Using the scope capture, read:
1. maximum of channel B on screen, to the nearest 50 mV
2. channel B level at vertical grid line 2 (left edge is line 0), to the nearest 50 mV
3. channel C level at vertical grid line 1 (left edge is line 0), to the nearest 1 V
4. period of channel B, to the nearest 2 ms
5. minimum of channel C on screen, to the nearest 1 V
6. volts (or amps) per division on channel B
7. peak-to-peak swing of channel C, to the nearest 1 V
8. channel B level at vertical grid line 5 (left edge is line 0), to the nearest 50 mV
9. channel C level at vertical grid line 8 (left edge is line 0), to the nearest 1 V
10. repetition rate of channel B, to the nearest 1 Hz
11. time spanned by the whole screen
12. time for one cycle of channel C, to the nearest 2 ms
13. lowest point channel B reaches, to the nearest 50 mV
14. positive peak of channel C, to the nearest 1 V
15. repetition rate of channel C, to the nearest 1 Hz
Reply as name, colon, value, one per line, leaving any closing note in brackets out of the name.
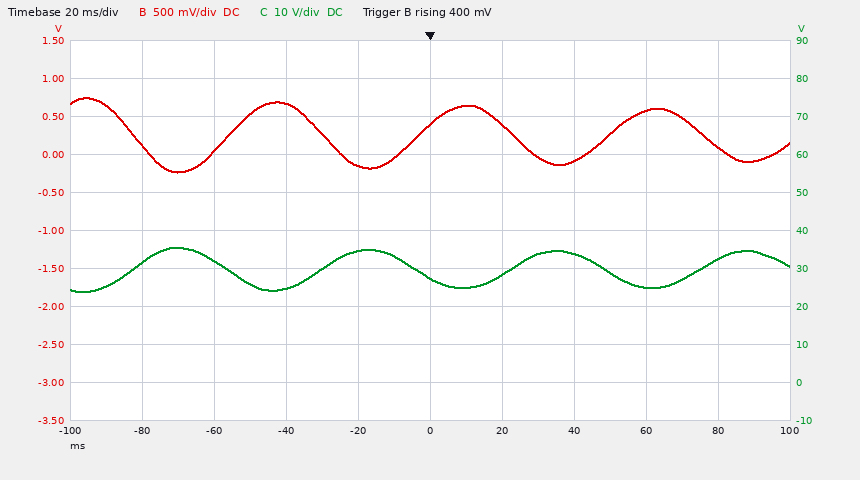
maximum of channel B on screen, to the nearest 50 mV: 750 mV
channel B level at vertical grid line 2 (left edge is line 0), to the nearest 50 mV: 50 mV
channel C level at vertical grid line 1 (left edge is line 0), to the nearest 1 V: 32 V
period of channel B, to the nearest 2 ms: 52 ms
minimum of channel C on screen, to the nearest 1 V: 24 V
volts (or amps) per division on channel B: 500 mV
peak-to-peak swing of channel C, to the nearest 1 V: 12 V
channel B level at vertical grid line 5 (left edge is line 0), to the nearest 50 mV: 400 mV
channel C level at vertical grid line 8 (left edge is line 0), to the nearest 1 V: 25 V
repetition rate of channel B, to the nearest 1 Hz: 19 Hz
time spanned by the whole screen: 200 ms
time for one cycle of channel C, to the nearest 2 ms: 52 ms
lowest point channel B reaches, to the nearest 50 mV: -250 mV
positive peak of channel C, to the nearest 1 V: 36 V
repetition rate of channel C, to the nearest 1 Hz: 19 Hz
